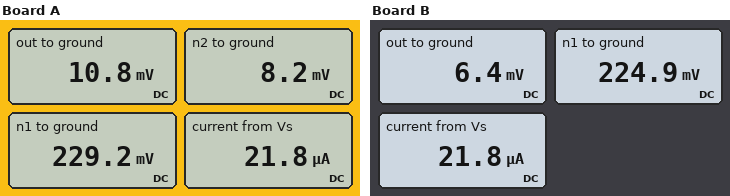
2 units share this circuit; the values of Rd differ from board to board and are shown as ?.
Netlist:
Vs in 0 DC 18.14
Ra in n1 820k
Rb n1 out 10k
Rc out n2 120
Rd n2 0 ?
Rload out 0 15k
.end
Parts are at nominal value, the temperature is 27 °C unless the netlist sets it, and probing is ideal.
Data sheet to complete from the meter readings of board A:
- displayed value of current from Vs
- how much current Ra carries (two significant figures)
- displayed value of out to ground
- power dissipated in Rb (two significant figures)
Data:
21.8 µA
22 µA
10.8 mV
4.8 µW
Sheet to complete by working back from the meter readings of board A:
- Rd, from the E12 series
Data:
390 Ω
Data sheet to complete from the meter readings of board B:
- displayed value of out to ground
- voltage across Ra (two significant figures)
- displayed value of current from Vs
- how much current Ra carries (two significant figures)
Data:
6.4 mV
18 V
21.8 µA
22 µA
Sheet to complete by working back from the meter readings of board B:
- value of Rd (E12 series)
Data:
180 Ω
